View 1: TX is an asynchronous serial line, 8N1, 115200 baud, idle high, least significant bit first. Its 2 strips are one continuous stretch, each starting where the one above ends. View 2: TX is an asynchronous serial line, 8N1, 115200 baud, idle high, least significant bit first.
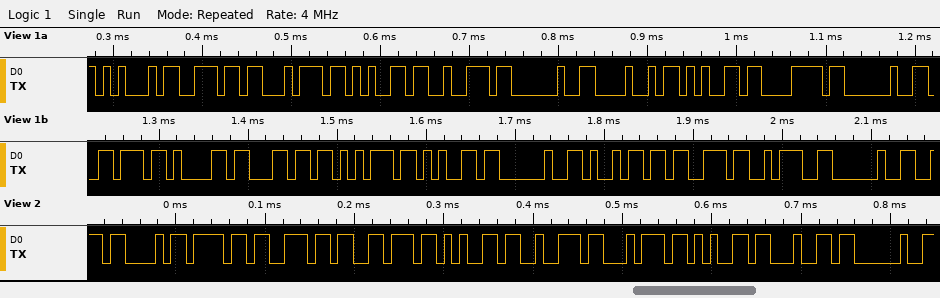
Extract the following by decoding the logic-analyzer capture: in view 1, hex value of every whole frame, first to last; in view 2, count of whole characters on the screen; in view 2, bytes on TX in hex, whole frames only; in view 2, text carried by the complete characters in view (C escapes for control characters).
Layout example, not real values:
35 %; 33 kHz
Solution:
45 6E 74 65 72 20 48 65 78 20 76 61 6C 75 65 20 69 73 3A 20; 10; 43 6F 6E 76 65 72 74 65 64 20; "Converted "
